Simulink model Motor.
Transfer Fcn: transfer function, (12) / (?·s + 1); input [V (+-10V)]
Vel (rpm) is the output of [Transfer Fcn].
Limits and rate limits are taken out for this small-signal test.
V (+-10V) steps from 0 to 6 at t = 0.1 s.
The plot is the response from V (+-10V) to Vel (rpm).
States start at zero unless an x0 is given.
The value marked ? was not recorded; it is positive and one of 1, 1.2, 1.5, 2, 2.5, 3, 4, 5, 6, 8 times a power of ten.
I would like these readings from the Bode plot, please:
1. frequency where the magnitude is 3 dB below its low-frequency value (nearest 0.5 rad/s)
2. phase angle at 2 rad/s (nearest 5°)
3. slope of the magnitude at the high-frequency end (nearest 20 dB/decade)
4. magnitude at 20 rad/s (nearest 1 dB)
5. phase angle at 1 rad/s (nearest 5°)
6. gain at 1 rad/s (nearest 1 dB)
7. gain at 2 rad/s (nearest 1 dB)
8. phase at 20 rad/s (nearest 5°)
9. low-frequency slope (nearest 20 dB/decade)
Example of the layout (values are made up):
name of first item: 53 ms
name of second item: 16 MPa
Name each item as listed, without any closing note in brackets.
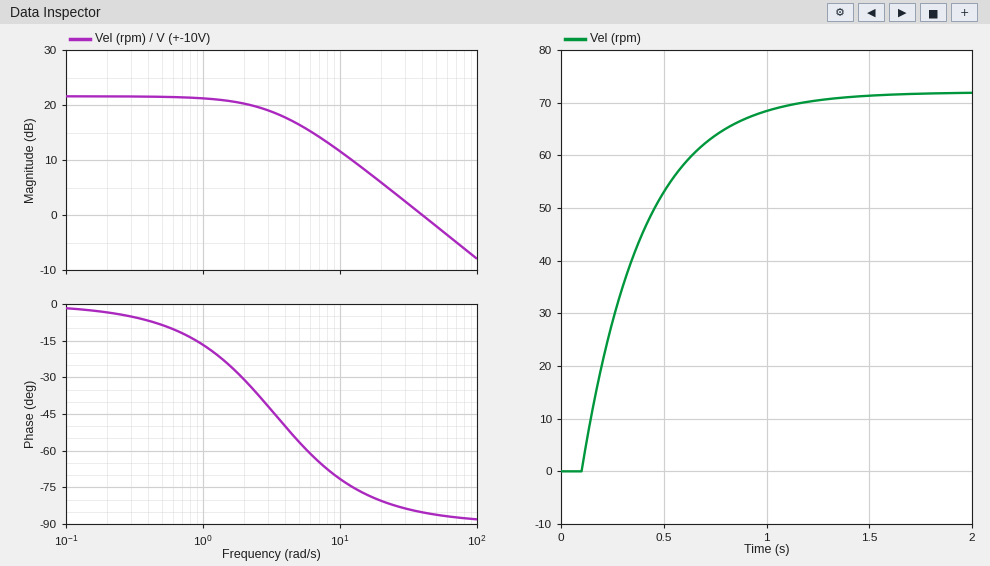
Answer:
frequency where the magnitude is 3 dB below its low-frequency value: 3.5 rad/s
phase angle at 2 rad/s: -30°
slope of the magnitude at the high-frequency end: -20 dB/decade
magnitude at 20 rad/s: 6 dB
phase angle at 1 rad/s: -15°
gain at 1 rad/s: 21 dB
gain at 2 rad/s: 20 dB
phase at 20 rad/s: -80°
low-frequency slope: 0 dB/decade
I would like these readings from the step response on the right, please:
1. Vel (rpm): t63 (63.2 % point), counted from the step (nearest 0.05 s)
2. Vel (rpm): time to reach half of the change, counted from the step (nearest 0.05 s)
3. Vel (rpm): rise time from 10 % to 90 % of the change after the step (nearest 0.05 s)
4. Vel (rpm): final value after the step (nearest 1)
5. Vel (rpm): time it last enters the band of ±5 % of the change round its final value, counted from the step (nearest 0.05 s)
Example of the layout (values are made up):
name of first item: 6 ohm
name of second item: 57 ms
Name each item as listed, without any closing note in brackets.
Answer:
Vel (rpm): t63 (63.2 % point), counted from the step: 0.30 s
Vel (rpm): time to reach half of the change, counted from the step: 0.20 s
Vel (rpm): rise time from 10 % to 90 % of the change after the step: 0.65 s
Vel (rpm): final value after the step: 72
Vel (rpm): time it last enters the band of ±5 % of the change round its final value, counted from the step: 0.90 s
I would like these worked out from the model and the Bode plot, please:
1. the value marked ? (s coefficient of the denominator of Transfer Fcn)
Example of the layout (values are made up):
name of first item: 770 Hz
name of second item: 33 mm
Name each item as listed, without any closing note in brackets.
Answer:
the value marked ?: 0.3
